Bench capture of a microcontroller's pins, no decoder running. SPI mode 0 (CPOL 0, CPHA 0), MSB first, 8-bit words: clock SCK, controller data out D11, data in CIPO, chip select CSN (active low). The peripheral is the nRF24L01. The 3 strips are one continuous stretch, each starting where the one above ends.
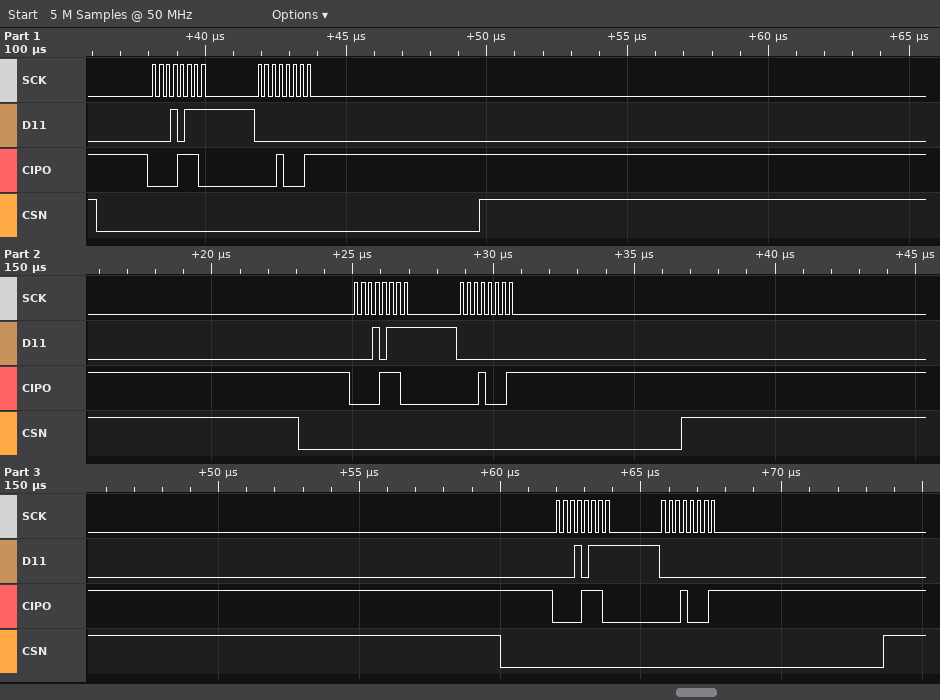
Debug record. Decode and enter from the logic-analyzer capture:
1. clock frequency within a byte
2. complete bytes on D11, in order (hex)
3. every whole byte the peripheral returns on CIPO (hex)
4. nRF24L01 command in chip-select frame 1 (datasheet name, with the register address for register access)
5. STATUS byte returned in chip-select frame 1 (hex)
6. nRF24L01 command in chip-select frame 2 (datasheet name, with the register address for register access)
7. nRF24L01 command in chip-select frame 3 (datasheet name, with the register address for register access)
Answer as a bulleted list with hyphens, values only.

- 4 MHz
- 0x17 0x00 0x17 0x00 0x17 0x00
- 0x0E 0x11 0x0E 0x11 0x0E 0x11
- R_REGISTER 0x17
- 0x0E
- R_REGISTER 0x17
- R_REGISTER 0x17
